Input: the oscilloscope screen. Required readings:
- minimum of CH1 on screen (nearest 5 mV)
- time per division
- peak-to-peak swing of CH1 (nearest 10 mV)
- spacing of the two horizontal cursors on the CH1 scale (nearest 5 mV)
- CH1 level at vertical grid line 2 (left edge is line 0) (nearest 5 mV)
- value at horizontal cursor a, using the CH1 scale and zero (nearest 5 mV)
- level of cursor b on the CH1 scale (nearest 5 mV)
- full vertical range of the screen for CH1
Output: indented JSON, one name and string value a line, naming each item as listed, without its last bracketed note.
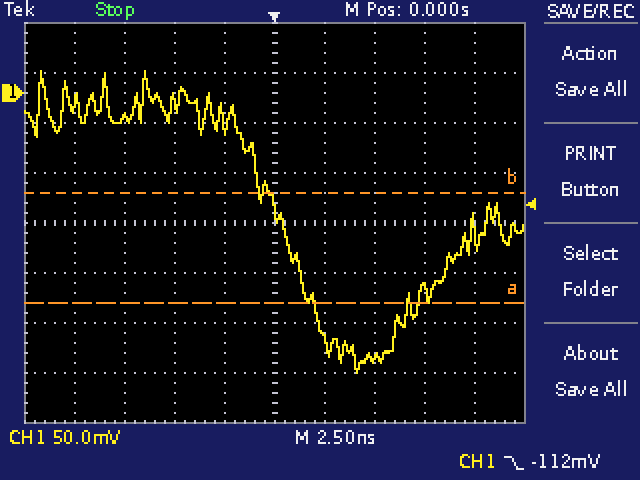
{
  "minimum of CH1 on screen": "-280 mV",
  "time per division": "2.5 ns",
  "peak-to-peak swing of CH1": "300 mV",
  "spacing of the two horizontal cursors on the CH1 scale": "110 mV",
  "CH1 level at vertical grid line 2 (left edge is line 0)": "-25 mV",
  "value at horizontal cursor a, using the CH1 scale and zero": "-210 mV",
  "level of cursor b on the CH1 scale": "-100 mV",
  "full vertical range of the screen for CH1": "400 mV"
}
